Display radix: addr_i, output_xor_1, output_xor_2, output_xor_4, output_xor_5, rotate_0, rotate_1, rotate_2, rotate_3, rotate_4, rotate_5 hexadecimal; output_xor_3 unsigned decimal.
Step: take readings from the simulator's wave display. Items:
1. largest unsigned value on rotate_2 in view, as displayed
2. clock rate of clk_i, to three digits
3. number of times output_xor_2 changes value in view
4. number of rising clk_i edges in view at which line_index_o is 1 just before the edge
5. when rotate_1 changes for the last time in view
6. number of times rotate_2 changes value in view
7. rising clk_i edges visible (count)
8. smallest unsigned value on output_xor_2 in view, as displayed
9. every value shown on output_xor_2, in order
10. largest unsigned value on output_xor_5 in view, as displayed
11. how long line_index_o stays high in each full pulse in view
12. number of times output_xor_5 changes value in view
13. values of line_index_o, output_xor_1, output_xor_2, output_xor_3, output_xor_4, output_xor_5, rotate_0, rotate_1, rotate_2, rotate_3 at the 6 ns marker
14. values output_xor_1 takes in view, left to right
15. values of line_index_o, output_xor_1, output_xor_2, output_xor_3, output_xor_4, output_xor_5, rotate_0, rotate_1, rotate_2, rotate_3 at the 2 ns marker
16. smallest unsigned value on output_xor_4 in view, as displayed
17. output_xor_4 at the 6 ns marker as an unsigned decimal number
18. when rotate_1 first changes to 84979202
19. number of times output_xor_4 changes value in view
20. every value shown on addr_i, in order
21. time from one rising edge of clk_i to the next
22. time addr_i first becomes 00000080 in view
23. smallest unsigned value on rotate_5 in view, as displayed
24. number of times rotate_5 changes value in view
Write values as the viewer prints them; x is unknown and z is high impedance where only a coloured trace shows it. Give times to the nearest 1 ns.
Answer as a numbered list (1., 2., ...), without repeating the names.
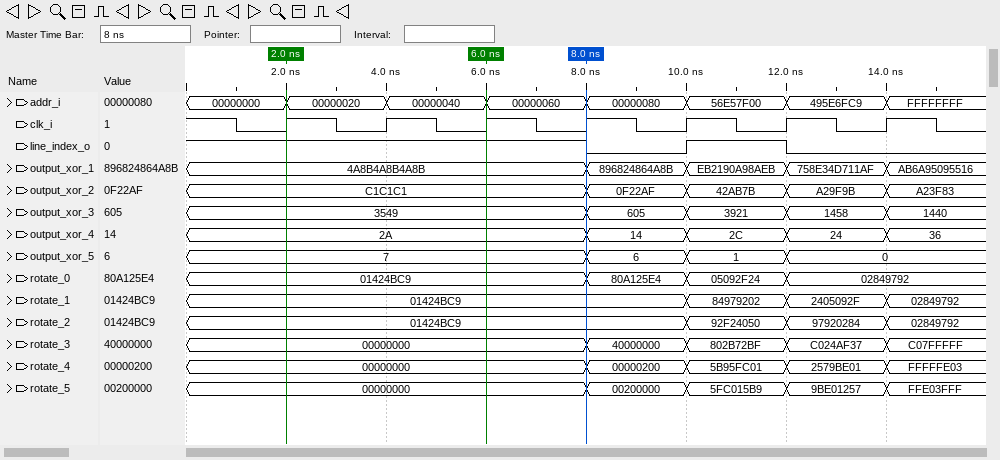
1. 97920284
2. 500 MHz
3. 4
4. 5
5. 14 ns
6. 3
7. 7
8. 0F22AF
9. C1C1C1, 0F22AF, 42AB7B, A29F9B, A23F83
10. 7
11. 2 ns
12. 3
13. line_index_o=1, output_xor_1=4A8B4A8B4A8B, output_xor_2=C1C1C1, output_xor_3=3549, output_xor_4=2A, output_xor_5=7, rotate_0=01424BC9, rotate_1=01424BC9, rotate_2=01424BC9, rotate_3=00000000
14. 4A8B4A8B4A8B, 896824864A8B, EB2190A98AEB, 758E34D711AF, AB6A95095516
15. line_index_o=1, output_xor_1=4A8B4A8B4A8B, output_xor_2=C1C1C1, output_xor_3=3549, output_xor_4=2A, output_xor_5=7, rotate_0=01424BC9, rotate_1=01424BC9, rotate_2=01424BC9, rotate_3=00000000
16. 14
17. 42
18. 10 ns
19. 4
20. 00000000, 00000020, 00000040, 00000060, 00000080, 56E57F00, 495E6FC9, FFFFFFFF
21. 2 ns
22. 8 ns
23. 00000000
24. 4
